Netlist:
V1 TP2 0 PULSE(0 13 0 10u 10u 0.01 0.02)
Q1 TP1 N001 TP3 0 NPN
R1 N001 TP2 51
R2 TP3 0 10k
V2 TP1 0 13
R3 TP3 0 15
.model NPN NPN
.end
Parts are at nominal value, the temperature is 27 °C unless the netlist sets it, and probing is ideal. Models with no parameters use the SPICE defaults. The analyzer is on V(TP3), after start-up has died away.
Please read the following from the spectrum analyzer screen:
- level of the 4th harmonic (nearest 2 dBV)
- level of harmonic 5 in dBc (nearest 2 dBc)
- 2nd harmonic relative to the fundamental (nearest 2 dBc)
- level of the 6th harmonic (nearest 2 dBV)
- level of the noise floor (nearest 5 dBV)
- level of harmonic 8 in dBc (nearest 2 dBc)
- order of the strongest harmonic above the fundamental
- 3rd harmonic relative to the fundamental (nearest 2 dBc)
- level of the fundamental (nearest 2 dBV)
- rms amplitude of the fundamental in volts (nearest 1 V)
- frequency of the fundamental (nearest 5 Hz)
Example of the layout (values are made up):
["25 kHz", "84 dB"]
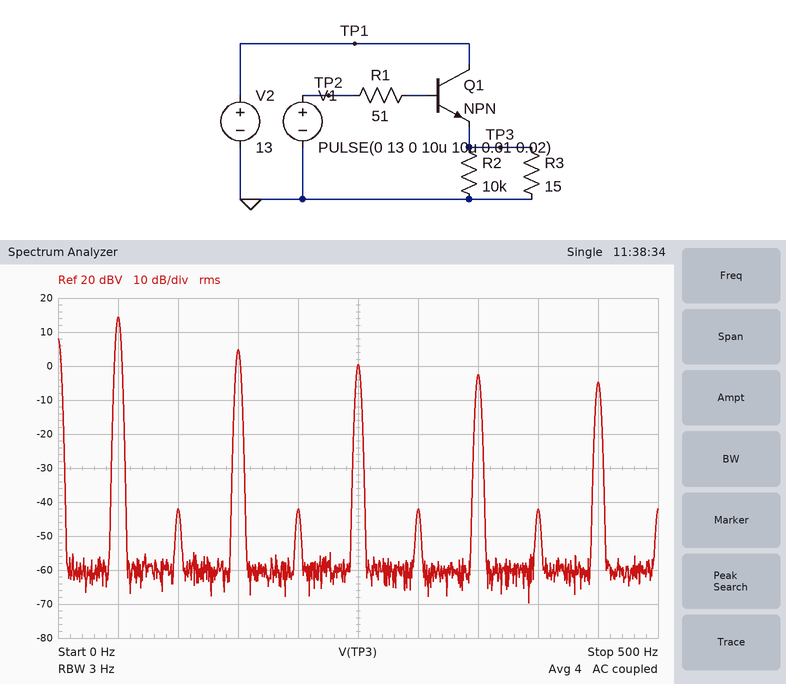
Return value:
["-42 dBV", "-14 dBc", "-56 dBc", "-42 dBV", "-60 dBV", "-56 dBc", "3", "-10 dBc", "14 dBV", "5 V", "50 Hz"]
